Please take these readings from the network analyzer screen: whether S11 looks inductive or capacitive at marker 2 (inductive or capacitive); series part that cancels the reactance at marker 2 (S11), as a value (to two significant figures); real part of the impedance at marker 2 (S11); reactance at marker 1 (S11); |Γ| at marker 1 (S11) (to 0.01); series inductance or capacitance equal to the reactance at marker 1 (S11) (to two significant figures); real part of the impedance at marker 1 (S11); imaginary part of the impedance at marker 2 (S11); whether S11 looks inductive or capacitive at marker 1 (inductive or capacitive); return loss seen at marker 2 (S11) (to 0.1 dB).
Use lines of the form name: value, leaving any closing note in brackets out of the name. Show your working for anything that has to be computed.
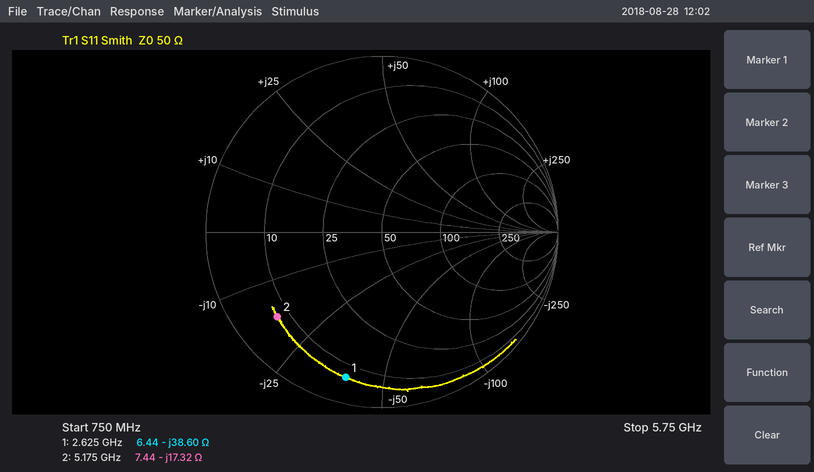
whether S11 looks inductive or capacitive at marker 2: capacitive
series part that cancels the reactance at marker 2 (S11), as a value: L = 17.32 Ω/(2π × 5.175 GHz) ≈ 533 pH, so 530 pH to two significant figures
real part of the impedance at marker 2: 7.44 Ω
reactance at marker 1: -38.60 Ω
|Γ| at marker 1 (S11): 0.85
series inductance or capacitance equal to the reactance at marker 1 (S11): C = 1/(2π × 2.625 GHz × 38.6 Ω) ≈ 1.6 pF
real part of the impedance at marker 1: 6.44 Ω
imaginary part of the impedance at marker 2: -17.32 Ω
whether S11 looks inductive or capacitive at marker 1: capacitive
return loss seen at marker 2 (S11): 2.3 dB
